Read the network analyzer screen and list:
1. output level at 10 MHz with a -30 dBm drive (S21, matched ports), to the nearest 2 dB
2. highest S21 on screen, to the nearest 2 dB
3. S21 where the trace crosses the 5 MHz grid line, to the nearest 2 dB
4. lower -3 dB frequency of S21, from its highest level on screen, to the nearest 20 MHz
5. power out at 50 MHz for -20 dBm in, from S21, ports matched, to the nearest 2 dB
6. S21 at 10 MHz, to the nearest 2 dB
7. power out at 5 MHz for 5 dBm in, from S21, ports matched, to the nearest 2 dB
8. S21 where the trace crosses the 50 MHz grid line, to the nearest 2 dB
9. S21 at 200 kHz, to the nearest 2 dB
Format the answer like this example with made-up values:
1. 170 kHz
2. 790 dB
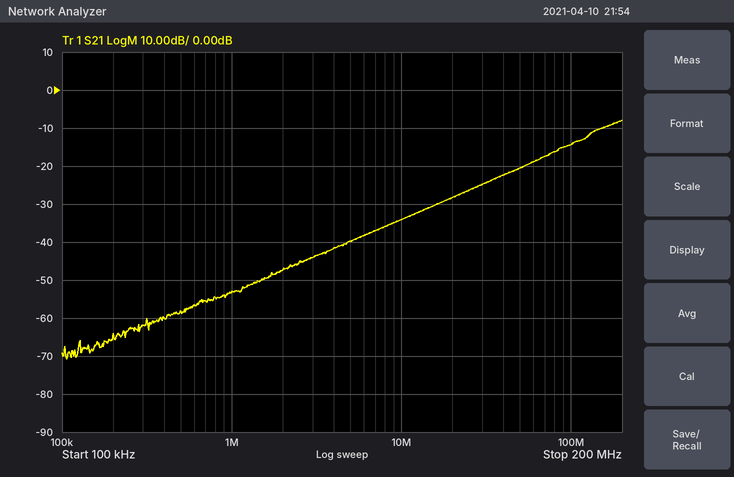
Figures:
1. -64 dBm
2. -8 dB
3. -40 dB
4. 140 MHz
5. -40 dBm
6. -34 dB
7. -34 dBm
8. -20 dB
9. -64 dB
